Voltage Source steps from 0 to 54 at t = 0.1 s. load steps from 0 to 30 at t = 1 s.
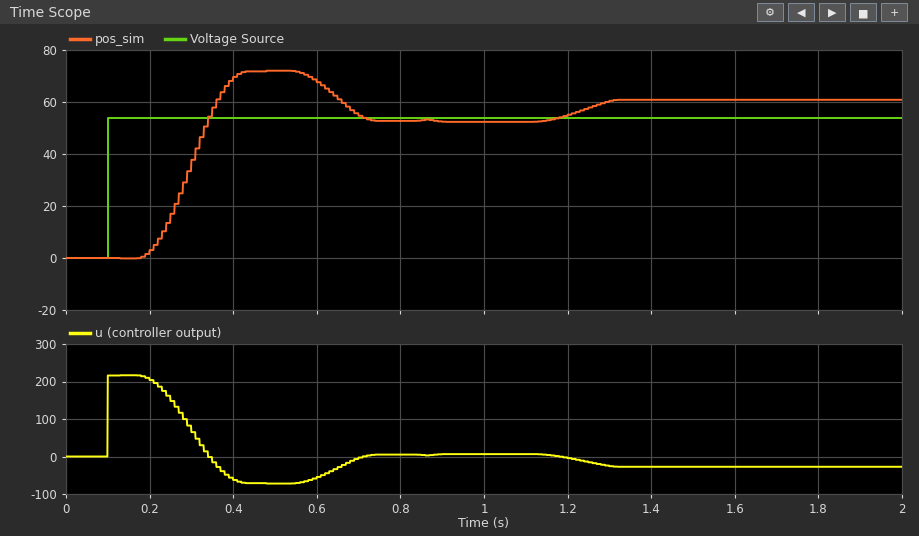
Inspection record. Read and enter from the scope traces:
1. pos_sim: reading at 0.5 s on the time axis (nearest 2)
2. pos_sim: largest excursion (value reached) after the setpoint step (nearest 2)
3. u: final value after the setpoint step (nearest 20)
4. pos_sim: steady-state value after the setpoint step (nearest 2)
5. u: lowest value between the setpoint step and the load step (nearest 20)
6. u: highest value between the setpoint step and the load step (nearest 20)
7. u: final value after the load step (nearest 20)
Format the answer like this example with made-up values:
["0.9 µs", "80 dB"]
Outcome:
["72", "72", "0", "52", "-80", "220", "-20"]
